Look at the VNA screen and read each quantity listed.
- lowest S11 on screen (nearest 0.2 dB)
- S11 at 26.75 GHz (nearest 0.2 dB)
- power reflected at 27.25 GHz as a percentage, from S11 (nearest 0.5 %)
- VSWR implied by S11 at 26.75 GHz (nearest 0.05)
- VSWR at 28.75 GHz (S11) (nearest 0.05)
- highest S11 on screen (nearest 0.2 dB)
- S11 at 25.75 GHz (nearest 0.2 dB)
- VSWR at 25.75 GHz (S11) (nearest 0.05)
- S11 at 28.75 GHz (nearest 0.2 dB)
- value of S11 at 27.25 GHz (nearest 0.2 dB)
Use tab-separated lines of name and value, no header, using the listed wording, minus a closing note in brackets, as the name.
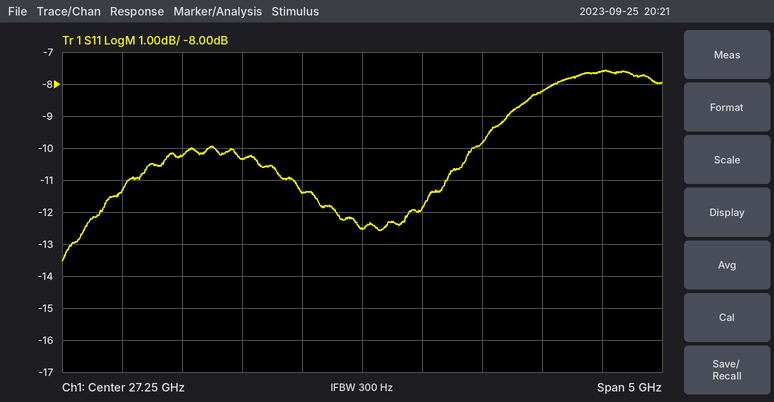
lowest S11 on screen	-13.6 dB
S11 at 26.75 GHz	-11.4 dB
power reflected at 27.25 GHz as a percentage, from S11	5.5 %
VSWR implied by S11 at 26.75 GHz	1.75
VSWR at 28.75 GHz (S11)	2.25
highest S11 on screen	-7.6 dB
S11 at 25.75 GHz	-10.2 dB
VSWR at 25.75 GHz (S11)	1.90
S11 at 28.75 GHz	-8.2 dB
value of S11 at 27.25 GHz	-12.6 dB
